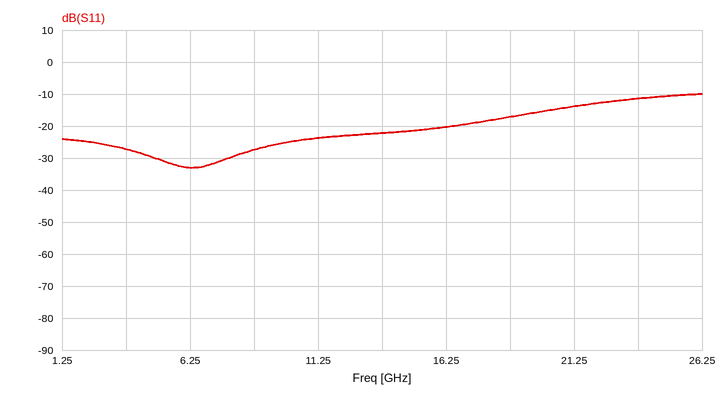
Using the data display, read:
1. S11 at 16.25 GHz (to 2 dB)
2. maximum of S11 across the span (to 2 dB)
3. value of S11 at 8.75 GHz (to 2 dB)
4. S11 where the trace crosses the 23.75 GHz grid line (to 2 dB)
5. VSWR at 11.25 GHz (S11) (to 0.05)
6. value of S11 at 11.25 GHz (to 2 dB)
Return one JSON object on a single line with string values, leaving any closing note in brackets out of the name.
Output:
{"S11 at 16.25 GHz": "-20 dB", "maximum of S11 across the span": "-10 dB", "value of S11 at 8.75 GHz": "-28 dB", "S11 where the trace crosses the 23.75 GHz grid line": "-12 dB", "VSWR at 11.25 GHz (S11)": "1.15", "value of S11 at 11.25 GHz": "-24 dB"}
